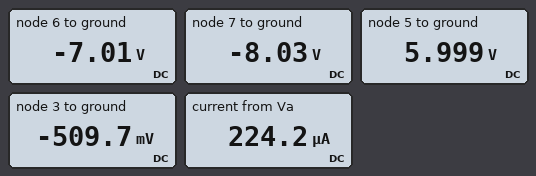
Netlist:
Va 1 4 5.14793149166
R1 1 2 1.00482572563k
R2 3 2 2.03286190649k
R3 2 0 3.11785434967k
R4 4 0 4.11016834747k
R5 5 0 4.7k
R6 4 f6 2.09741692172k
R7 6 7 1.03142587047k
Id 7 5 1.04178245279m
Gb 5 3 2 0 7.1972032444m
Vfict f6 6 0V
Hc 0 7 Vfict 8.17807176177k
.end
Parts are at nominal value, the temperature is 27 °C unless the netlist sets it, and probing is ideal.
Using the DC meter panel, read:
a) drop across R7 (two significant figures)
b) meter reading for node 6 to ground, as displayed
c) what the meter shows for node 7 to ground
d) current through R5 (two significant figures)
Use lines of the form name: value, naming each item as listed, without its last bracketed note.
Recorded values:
drop across R7: 1.0 V
meter reading for node 6 to ground, as displayed: -7.01 V
what the meter shows for node 7 to ground: -8.03 V
current through R5: 1.3 mA
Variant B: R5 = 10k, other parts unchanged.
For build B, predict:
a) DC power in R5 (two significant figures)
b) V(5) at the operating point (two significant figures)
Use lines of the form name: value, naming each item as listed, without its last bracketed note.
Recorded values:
DC power in R5: 16 mW
V(5) at the operating point: 13 V
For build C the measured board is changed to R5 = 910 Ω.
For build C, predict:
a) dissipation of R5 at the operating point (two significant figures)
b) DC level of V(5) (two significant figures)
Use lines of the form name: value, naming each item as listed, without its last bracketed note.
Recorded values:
dissipation of R5 at the operating point: 1.5 mW
DC level of V(5): 1.2 V
